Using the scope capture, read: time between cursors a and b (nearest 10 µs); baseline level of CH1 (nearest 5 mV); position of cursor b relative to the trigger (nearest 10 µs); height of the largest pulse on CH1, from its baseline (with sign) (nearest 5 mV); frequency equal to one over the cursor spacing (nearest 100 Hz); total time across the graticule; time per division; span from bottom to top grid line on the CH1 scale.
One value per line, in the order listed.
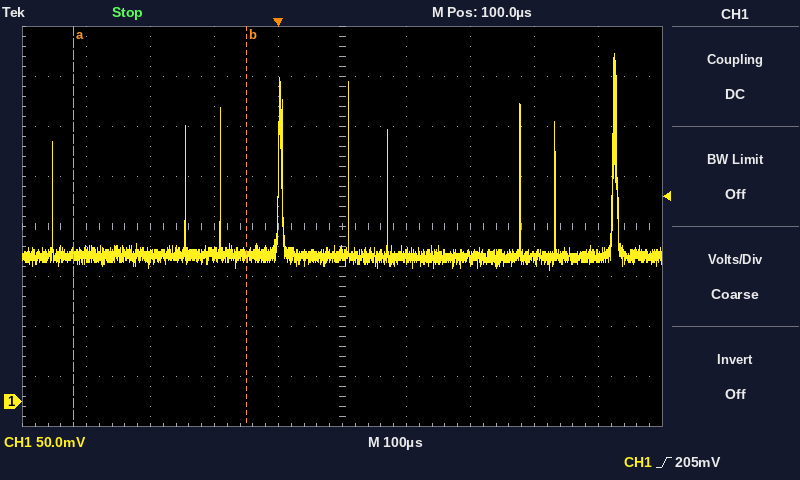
270 µs
145 mV
-50 µs
+200 mV
3.7 kHz
1 ms
100 µs
400 mV
